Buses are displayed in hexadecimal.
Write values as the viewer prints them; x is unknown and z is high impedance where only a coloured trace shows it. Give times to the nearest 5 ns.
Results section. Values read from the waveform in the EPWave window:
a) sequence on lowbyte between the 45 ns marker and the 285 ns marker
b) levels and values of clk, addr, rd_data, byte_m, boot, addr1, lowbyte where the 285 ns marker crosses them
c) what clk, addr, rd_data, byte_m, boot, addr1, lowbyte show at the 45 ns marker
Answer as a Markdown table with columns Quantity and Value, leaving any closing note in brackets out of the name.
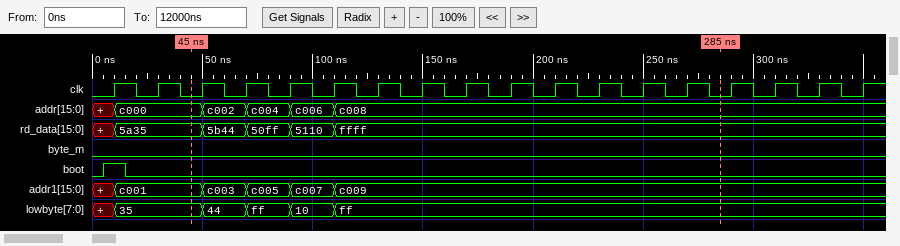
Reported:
| Quantity | Value |
|---|---|
| sequence on lowbyte between the 45 ns marker and the 285 ns marker | 35, 44, ff, 10, ff |
| levels and values of clk, addr, rd_data, byte_m, boot, addr1, lowbyte where the 285 ns marker crosses them | clk=0, addr=c008, rd_data=ffff, byte_m=0, boot=0, addr1=c009, lowbyte=ff |
| what clk, addr, rd_data, byte_m, boot, addr1, lowbyte show at the 45 ns marker | clk=0, addr=c000, rd_data=5a35, byte_m=0, boot=0, addr1=c001, lowbyte=35 |
